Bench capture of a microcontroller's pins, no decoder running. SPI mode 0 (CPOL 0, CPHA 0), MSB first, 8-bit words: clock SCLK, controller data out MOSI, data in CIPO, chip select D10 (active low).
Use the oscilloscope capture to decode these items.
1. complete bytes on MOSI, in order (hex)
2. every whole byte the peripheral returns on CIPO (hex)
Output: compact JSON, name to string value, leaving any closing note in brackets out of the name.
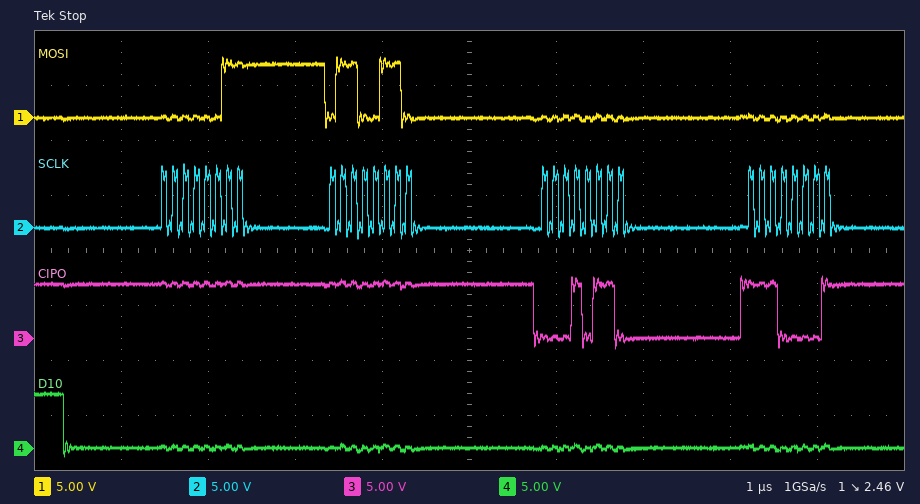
{"complete bytes on MOSI, in order": "0x03 0x66 0x00 0x00", "every whole byte the peripheral returns on CIPO": "0xFF 0xFF 0x16 0xE1"}
